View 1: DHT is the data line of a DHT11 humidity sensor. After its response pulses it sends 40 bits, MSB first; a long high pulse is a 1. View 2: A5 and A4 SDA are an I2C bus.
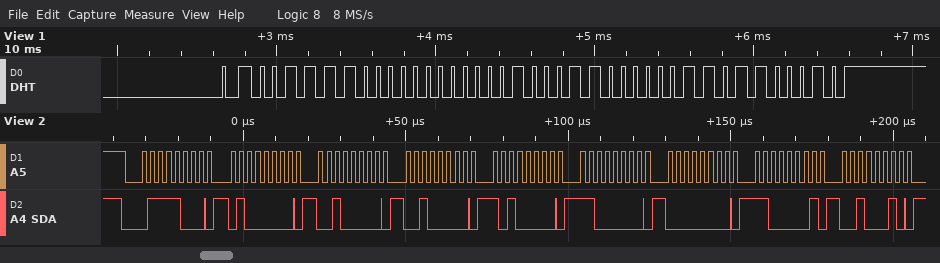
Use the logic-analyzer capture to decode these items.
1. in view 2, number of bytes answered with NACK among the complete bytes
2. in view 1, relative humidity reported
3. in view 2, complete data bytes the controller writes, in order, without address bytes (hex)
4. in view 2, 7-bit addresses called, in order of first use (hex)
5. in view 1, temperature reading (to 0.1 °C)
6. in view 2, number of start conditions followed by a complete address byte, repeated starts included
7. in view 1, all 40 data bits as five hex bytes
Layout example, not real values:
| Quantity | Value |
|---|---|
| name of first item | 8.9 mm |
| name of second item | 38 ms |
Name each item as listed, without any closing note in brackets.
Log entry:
| Quantity | Value |
|---|---|
| in view 2, number of bytes answered with NACK among the complete bytes | 0 |
| in view 1, relative humidity reported | 60 % |
| in view 2, complete data bytes the controller writes, in order, without address bytes | 40 20 20 A0 C0 00 C1 22 |
| in view 2, 7-bit addresses called, in order of first use | 0x3C |
| in view 1, temperature reading | 35.3 °C |
| in view 2, number of start conditions followed by a complete address byte, repeated starts included | 1 |
| in view 1, all 40 data bits as five hex bytes | 3C 00 23 03 62 |
